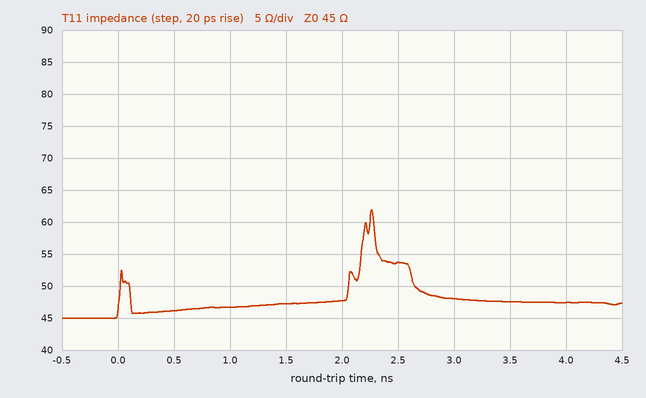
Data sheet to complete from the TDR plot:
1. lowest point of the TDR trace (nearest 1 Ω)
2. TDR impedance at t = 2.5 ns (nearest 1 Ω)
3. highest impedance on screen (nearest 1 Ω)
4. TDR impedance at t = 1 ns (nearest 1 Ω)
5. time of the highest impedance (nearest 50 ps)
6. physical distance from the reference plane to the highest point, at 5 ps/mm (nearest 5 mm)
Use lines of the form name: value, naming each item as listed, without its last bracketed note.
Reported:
lowest point of the TDR trace: 45 Ω
TDR impedance at t = 2.5 ns: 54 Ω
highest impedance on screen: 62 Ω
TDR impedance at t = 1 ns: 47 Ω
time of the highest impedance: 2.25 ns
physical distance from the reference plane to the highest point, at 5 ps/mm: 225 mm
